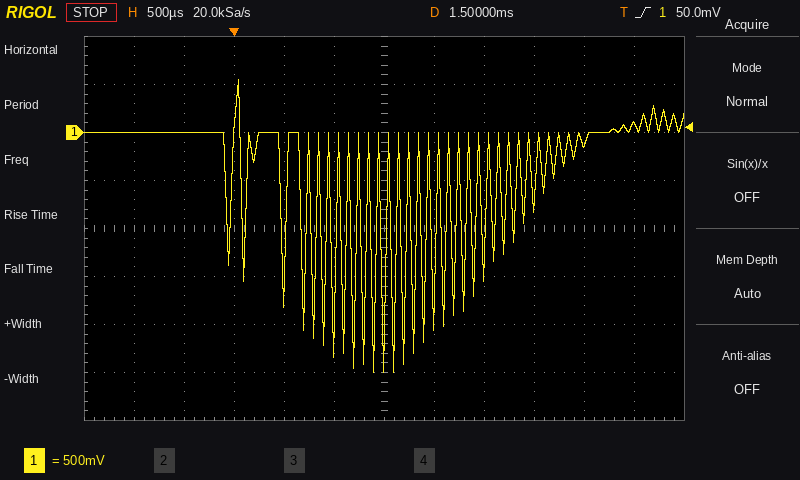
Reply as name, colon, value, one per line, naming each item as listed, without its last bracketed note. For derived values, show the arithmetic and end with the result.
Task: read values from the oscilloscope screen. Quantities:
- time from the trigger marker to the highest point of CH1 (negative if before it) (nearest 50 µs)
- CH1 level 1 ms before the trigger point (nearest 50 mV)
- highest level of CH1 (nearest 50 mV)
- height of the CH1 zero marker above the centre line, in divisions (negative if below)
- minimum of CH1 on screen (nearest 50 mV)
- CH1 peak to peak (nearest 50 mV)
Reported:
time from the trigger marker to the highest point of CH1 (negative if before it): +50 µs
CH1 level 1 ms before the trigger point: 0 mV
highest level of CH1: 550 mV
height of the CH1 zero marker above the centre line, in divisions: +2.0 div
minimum of CH1 on screen: -2.50 V
CH1 peak to peak: 550 mV − (-2.50 V) = 3.05 V
